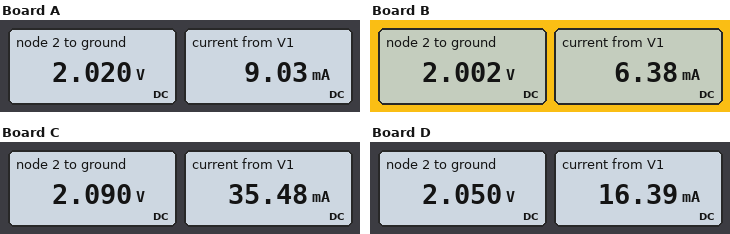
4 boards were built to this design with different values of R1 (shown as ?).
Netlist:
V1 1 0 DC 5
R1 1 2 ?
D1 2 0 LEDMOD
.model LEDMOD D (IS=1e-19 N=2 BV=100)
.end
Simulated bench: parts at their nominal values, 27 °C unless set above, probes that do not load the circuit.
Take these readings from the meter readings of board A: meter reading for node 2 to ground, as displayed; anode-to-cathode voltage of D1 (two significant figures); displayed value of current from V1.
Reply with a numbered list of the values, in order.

1. 2.020 V
2. 2.0 V
3. 9.03 mA
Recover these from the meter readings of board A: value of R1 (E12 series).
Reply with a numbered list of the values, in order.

1. 330 Ω
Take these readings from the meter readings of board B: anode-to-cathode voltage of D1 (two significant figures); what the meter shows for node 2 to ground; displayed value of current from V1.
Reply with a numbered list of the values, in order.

1. 2.0 V
2. 2.002 V
3. 6.38 mA
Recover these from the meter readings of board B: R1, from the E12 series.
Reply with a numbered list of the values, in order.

1. 470 Ω
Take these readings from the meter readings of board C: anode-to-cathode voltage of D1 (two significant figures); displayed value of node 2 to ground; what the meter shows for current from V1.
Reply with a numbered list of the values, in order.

1. 2.1 V
2. 2.090 V
3. 35.48 mA
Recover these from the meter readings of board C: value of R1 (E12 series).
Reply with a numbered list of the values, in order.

1. 82 Ω
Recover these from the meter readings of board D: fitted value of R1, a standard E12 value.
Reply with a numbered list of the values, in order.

1. 180 Ω
